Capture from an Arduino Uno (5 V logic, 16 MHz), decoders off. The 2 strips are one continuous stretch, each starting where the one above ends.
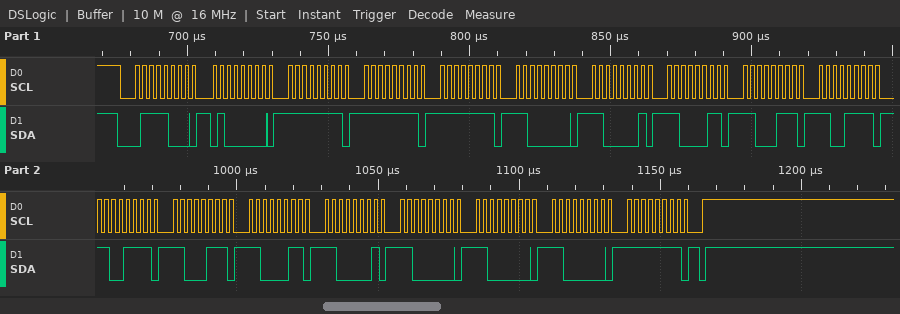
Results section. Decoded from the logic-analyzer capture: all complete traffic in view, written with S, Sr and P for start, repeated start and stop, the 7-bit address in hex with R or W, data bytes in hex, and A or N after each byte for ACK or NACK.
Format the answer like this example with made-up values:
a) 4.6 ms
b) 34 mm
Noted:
a) S 3CW A 40 A FF A FF A FF A C0 A C1 A C3 A C7 A CF A CF A C7 A C3 A C1 A C0 A C0 A C0 A FF A P
